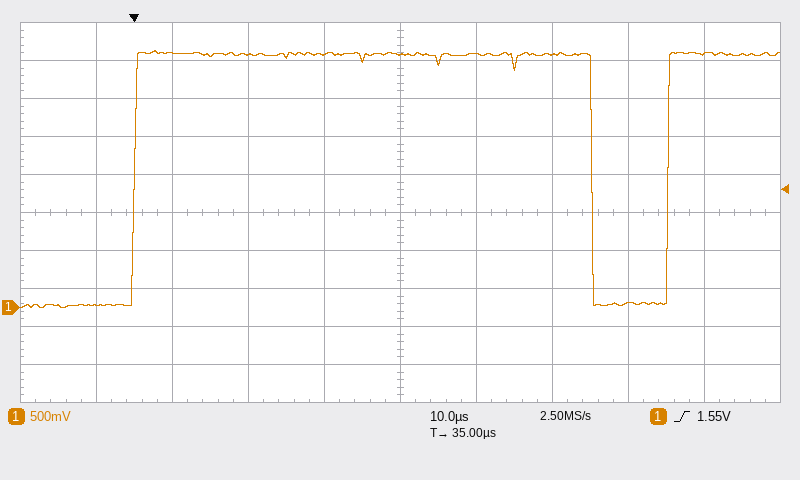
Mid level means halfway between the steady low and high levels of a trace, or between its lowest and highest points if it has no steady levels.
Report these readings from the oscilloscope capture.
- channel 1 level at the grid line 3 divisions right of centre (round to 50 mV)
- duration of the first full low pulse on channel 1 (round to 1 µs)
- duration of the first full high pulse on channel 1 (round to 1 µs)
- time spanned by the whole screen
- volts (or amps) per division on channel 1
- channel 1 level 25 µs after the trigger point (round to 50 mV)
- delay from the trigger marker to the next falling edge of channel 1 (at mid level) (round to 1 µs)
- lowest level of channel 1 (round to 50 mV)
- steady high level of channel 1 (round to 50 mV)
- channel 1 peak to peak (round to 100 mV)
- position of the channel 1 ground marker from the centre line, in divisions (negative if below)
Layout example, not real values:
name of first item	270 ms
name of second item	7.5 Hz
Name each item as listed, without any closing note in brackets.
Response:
channel 1 level at the grid line 3 divisions right of centre	50 mV
duration of the first full low pulse on channel 1	10 µs
duration of the first full high pulse on channel 1	60 µs
time spanned by the whole screen	100 µs
volts (or amps) per division on channel 1	500 mV
channel 1 level 25 µs after the trigger point	3.35 V
delay from the trigger marker to the next falling edge of channel 1 (at mid level)	60 µs
lowest level of channel 1	0 mV
steady high level of channel 1	3.35 V
channel 1 peak to peak	3.40 V
position of the channel 1 ground marker from the centre line, in divisions	-2.5 div
